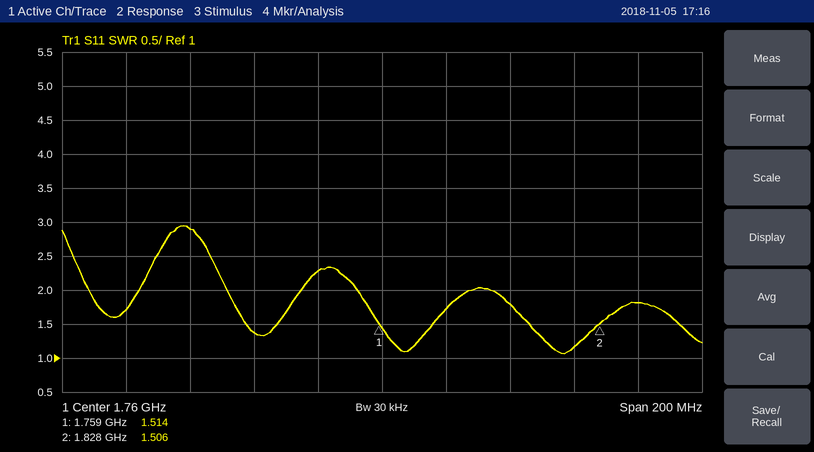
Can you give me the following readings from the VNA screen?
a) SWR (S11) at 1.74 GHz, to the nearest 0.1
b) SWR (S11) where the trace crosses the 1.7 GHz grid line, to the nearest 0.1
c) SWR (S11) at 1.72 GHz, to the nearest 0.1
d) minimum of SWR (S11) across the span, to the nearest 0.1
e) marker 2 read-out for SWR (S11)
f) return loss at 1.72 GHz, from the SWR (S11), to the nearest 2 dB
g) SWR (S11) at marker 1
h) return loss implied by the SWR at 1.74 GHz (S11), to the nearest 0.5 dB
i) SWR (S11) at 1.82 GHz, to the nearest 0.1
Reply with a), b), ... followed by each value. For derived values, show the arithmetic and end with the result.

a) 2.3
b) 2.9
c) 1.4
d) 1.1
e) 1.506
f) −20 log10((1.4 − 1)/(1.4 + 1)) ≈ 16 dB
g) 1.514
h) −20 log10((2.3 − 1)/(2.3 + 1)) ≈ 8.09 dB, so 8.0 dB to the nearest 0.5 dB
i) 1.2
